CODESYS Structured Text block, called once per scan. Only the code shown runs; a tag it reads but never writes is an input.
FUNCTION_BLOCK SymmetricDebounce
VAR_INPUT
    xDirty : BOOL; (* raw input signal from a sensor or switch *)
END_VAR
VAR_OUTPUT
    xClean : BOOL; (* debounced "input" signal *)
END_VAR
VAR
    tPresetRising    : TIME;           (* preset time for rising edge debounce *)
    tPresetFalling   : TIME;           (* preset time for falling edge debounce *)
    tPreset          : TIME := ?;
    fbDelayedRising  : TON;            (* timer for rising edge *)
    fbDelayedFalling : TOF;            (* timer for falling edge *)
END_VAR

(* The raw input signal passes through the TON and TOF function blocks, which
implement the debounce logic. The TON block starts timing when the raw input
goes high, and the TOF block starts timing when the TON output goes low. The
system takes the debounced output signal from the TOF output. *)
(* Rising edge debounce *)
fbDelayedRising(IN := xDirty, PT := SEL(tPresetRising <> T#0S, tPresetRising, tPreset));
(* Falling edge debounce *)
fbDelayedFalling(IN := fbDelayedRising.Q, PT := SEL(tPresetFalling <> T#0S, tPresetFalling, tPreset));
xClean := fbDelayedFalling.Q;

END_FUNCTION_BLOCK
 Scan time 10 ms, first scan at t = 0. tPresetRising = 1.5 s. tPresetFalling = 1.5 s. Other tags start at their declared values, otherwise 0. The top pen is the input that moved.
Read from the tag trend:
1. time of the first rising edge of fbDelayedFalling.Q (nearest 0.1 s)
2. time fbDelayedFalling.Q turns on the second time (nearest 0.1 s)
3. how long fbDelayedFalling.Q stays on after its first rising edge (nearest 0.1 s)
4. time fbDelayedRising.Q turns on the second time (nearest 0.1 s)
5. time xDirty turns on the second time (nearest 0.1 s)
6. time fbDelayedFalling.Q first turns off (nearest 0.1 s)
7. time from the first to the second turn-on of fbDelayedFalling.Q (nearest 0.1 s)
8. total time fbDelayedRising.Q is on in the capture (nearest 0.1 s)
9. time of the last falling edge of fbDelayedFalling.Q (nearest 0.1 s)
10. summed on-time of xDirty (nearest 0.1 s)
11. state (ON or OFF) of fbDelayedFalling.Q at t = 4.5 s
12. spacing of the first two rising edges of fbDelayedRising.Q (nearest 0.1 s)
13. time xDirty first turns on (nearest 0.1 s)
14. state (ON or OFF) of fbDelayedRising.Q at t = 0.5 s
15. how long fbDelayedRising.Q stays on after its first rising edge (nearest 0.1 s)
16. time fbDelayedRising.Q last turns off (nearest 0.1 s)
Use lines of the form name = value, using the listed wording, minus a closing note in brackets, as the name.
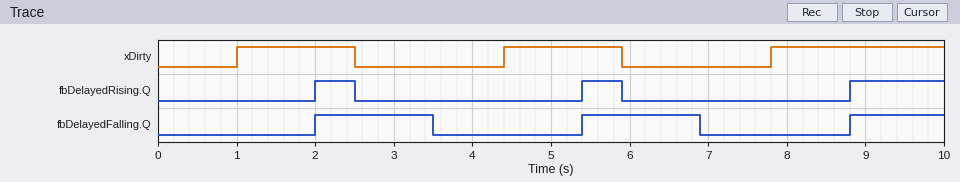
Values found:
time of the first rising edge of fbDelayedFalling.Q = 2.0 s
time fbDelayedFalling.Q turns on the second time = 5.4 s
how long fbDelayedFalling.Q stays on after its first rising edge = 1.5 s
time fbDelayedRising.Q turns on the second time = 5.4 s
time xDirty turns on the second time = 4.4 s
time fbDelayedFalling.Q first turns off = 3.5 s
time from the first to the second turn-on of fbDelayedFalling.Q = 3.4 s
total time fbDelayedRising.Q is on in the capture = 2.2 s
time of the last falling edge of fbDelayedFalling.Q = 6.9 s
summed on-time of xDirty = 5.2 s
state (ON or OFF) of fbDelayedFalling.Q at t = 4.5 s = OFF
spacing of the first two rising edges of fbDelayedRising.Q = 3.4 s
time xDirty first turns on = 1.0 s
state (ON or OFF) of fbDelayedRising.Q at t = 0.5 s = OFF
how long fbDelayedRising.Q stays on after its first rising edge = 0.5 s
time fbDelayedRising.Q last turns off = 5.9 s
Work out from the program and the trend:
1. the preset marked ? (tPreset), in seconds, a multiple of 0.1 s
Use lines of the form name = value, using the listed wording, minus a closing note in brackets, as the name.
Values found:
the preset marked ? (tPreset), in seconds, a multiple of 0.1 s = 1.0 s
